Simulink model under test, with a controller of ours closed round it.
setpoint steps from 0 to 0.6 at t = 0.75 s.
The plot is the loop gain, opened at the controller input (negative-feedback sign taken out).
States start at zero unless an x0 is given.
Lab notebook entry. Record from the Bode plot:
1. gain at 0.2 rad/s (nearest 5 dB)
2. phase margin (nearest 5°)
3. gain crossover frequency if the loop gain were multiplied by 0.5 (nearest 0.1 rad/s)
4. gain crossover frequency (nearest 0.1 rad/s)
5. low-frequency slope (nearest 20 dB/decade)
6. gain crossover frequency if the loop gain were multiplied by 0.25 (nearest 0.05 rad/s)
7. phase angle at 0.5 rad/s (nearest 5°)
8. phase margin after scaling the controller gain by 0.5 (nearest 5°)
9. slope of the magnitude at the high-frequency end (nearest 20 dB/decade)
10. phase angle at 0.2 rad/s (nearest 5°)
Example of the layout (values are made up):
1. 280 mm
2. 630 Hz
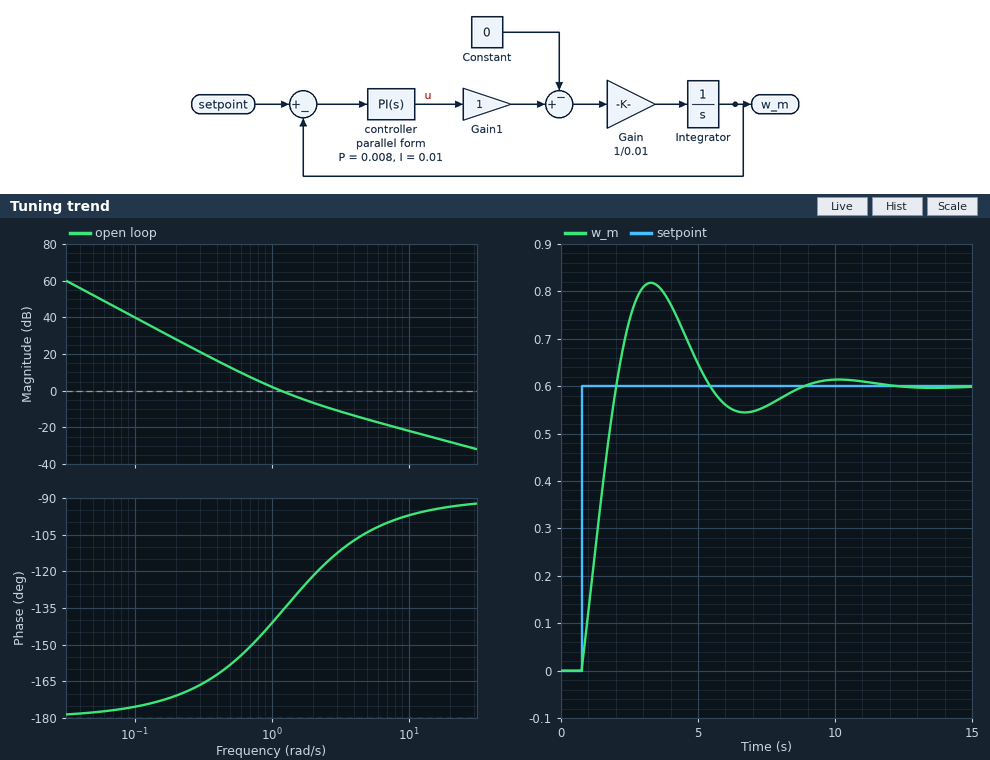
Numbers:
1. 30 dB
2. 45°
3. 0.8 rad/s
4. 1.2 rad/s
5. -40 dB/decade
6. 0.50 rad/s
7. -160°
8. 30°
9. -20 dB/decade
10. -170°
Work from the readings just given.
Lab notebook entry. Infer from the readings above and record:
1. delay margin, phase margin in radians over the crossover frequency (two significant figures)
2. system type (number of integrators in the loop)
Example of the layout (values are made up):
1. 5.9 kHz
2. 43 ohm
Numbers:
1. 0.65 s
2. 2
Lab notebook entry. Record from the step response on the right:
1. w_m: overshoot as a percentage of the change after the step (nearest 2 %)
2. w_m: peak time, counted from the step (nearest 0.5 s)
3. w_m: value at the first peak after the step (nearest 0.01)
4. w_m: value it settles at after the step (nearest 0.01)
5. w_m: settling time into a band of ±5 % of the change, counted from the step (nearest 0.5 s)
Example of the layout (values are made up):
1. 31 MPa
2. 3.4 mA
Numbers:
1. 36 %
2. 2.5 s
3. 0.82
4. 0.60
5. 7.0 s
